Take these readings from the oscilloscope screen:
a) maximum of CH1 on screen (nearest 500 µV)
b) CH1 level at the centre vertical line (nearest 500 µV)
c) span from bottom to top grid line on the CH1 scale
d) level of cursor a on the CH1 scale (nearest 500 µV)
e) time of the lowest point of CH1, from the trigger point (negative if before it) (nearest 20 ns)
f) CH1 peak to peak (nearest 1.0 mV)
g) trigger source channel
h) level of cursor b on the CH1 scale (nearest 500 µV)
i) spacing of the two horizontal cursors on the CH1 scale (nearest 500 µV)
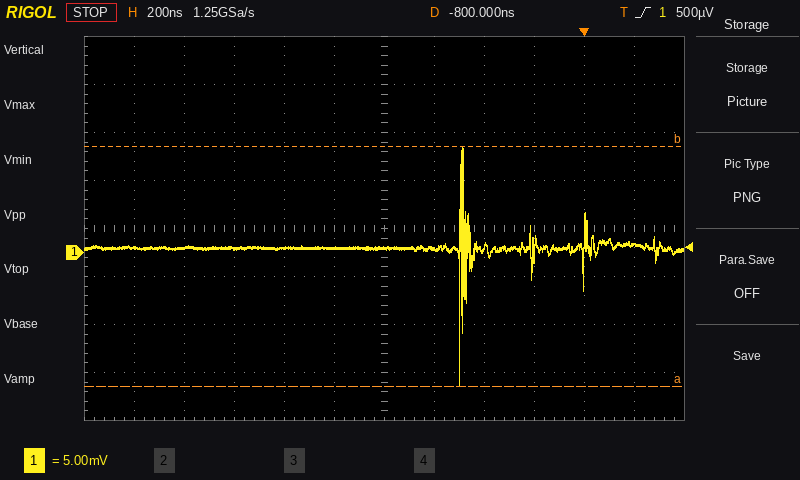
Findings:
11.0 mV
500 µV
40 mV
-14.0 mV
-500 ns
25.0 mV
CH1
11.0 mV
25.0 mV
